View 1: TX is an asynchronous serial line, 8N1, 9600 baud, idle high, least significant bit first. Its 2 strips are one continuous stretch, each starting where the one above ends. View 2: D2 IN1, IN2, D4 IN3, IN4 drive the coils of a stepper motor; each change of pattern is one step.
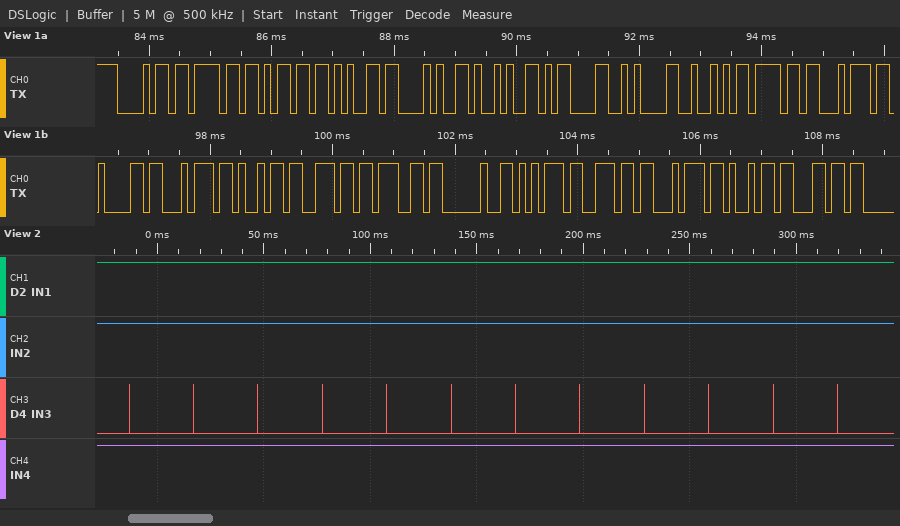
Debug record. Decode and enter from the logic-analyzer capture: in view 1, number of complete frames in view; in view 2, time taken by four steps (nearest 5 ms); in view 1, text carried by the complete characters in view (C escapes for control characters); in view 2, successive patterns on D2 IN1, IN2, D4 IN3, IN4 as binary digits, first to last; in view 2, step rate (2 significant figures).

22
120 ms
"home()\r\nRotating until"
1101 1101 1101 1101 1101 1101 1101 1101 1101 1101 1101 1101 1101
33 steps/s
